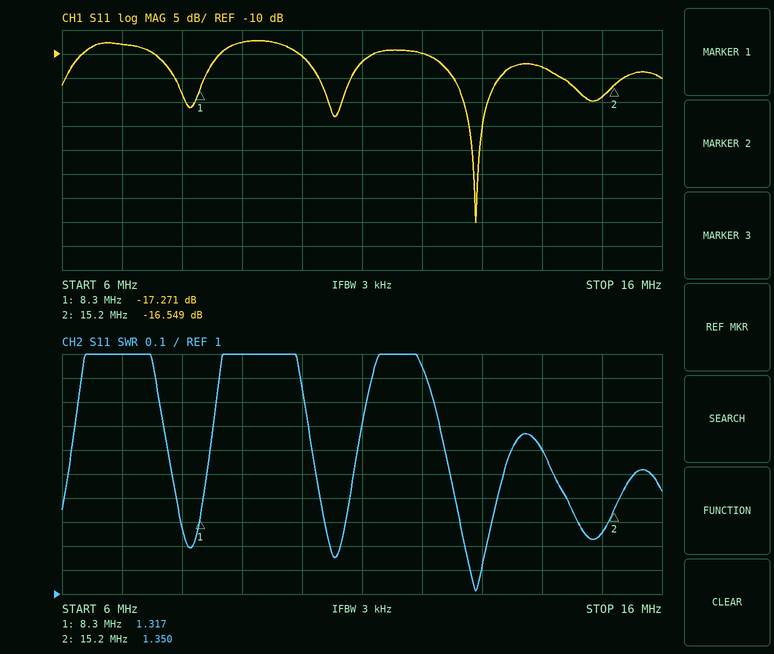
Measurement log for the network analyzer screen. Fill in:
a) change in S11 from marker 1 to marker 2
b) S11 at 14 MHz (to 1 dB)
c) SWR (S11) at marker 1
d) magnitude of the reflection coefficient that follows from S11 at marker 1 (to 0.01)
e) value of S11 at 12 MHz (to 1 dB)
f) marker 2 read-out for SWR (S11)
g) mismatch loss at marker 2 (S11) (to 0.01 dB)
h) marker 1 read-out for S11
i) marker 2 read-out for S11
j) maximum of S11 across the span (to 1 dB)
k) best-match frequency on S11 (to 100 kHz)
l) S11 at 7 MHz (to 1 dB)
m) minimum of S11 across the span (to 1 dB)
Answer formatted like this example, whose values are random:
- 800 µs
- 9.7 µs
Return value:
- 0.722 dB
- -13 dB
- 1.317
- 0.14
- -10 dB
- 1.350
- 0.10 dB
- -17.271 dB
- -16.549 dB
- -7 dB
- 12.9 MHz
- -8 dB
- -45 dB
